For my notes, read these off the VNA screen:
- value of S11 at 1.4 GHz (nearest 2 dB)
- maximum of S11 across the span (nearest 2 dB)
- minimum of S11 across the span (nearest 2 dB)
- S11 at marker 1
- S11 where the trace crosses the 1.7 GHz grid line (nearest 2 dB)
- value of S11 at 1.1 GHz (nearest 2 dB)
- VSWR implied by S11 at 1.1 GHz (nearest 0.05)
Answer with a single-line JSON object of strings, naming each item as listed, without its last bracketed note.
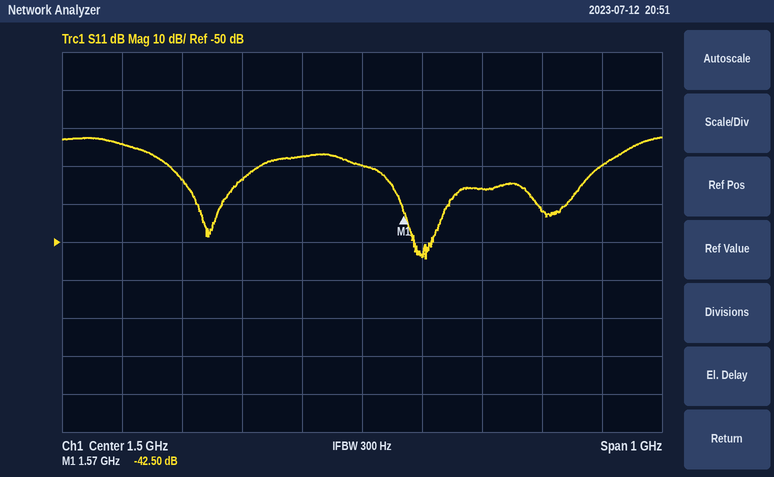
{"value of S11 at 1.4 GHz": "-28 dB", "maximum of S11 across the span": "-22 dB", "minimum of S11 across the span": "-54 dB", "S11 at marker 1": "-42.50 dB", "S11 where the trace crosses the 1.7 GHz grid line": "-36 dB", "value of S11 at 1.1 GHz": "-24 dB", "VSWR implied by S11 at 1.1 GHz": "1.15"}
